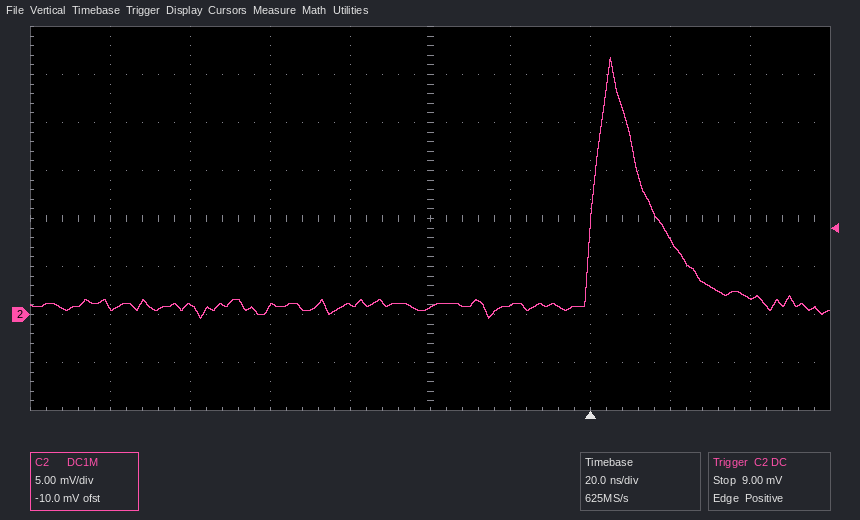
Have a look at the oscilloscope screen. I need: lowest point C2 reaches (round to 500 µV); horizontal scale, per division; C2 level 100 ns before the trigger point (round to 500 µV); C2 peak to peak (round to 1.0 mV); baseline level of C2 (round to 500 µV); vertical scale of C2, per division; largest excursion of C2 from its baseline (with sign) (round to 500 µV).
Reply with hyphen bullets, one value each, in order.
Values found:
- -500 µV
- 20 ns
- 1.0 mV
- 27.0 mV
- 1.0 mV
- 5 mV
- +26.0 mV
